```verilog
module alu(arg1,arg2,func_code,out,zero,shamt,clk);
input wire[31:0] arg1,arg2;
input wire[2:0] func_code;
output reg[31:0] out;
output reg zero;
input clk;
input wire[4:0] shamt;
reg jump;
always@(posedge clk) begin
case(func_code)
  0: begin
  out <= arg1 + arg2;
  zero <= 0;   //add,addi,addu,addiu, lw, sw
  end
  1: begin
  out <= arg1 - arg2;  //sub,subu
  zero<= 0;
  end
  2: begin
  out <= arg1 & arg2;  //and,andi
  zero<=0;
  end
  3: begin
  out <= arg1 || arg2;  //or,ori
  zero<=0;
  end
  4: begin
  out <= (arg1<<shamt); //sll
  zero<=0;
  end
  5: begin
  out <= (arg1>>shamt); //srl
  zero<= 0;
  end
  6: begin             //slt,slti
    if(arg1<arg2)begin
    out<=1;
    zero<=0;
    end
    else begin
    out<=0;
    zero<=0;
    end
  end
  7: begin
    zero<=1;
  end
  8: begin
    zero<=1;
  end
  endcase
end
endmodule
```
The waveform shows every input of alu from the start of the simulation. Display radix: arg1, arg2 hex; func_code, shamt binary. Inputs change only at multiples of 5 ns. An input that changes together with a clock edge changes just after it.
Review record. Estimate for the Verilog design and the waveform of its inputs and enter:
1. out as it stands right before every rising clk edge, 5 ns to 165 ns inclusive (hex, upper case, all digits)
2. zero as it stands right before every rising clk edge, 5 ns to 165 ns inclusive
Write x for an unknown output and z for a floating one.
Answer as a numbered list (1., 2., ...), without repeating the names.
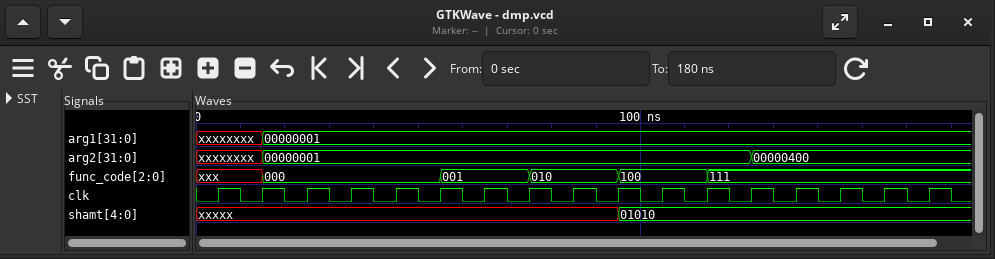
1. x, x, x, 00000002, 00000002, 00000002, 00000002, 00000000, 00000000, 00000001, 00000001, 00000400, 00000400, 00000400, 00000400, 00000400, 00000400
2. x x x 0 0 0 0 0 0 0 0 0 0 1 1 1 1
